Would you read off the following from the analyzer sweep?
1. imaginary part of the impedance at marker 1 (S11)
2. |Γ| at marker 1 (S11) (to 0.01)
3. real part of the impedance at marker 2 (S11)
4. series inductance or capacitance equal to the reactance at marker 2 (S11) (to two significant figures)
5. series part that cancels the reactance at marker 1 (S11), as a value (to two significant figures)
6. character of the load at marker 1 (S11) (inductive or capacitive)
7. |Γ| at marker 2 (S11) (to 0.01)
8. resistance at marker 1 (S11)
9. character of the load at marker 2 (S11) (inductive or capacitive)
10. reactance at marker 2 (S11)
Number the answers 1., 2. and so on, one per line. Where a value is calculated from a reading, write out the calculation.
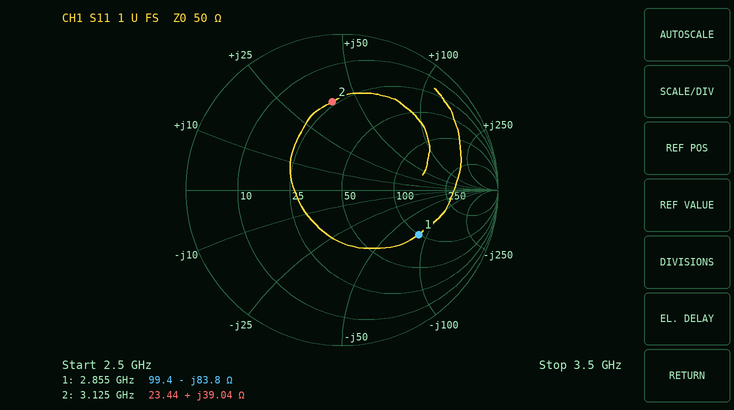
1. -83.8 Ω
2. 0.57
3. 23.44 Ω
4. L = 39.04 Ω/(2π × 3.125 GHz) ≈ 2.0 nH
5. L = 83.8 Ω/(2π × 2.855 GHz) ≈ 4.7 nH
6. capacitive
7. 0.57
8. 99.4 Ω
9. inductive
10. +39.04 Ω
